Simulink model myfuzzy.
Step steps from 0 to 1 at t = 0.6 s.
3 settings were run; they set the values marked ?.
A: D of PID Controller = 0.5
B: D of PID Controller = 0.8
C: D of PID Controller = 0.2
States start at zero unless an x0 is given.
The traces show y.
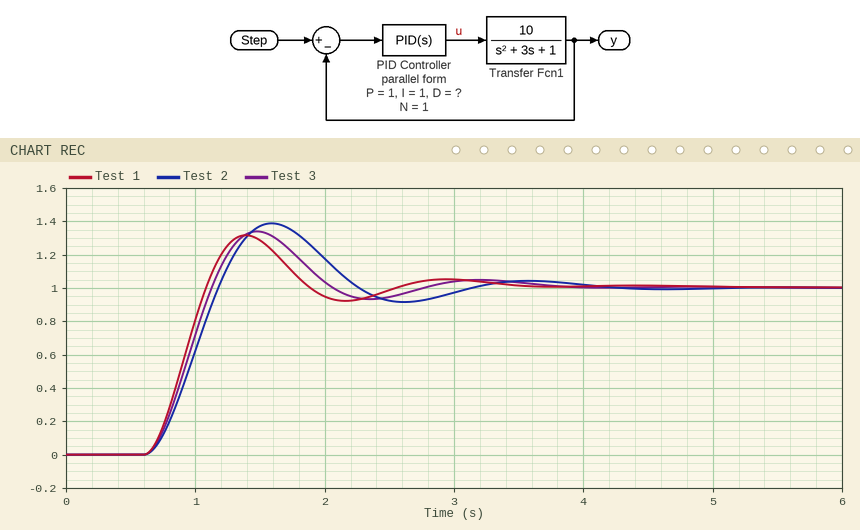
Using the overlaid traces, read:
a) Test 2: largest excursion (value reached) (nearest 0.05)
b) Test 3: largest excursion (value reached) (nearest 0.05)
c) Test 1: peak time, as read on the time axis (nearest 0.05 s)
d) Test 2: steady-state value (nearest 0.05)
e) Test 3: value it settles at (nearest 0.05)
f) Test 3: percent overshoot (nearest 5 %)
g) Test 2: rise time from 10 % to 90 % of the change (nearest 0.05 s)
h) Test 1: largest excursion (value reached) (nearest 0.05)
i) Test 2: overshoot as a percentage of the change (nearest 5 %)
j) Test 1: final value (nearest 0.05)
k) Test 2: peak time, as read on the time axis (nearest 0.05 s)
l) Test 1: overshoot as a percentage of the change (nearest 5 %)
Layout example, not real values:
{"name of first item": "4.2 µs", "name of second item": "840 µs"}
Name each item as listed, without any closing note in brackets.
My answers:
{"Test 2: largest excursion (value reached)": "1.40", "Test 3: largest excursion (value reached)": "1.35", "Test 1: peak time, as read on the time axis": "1.40 s", "Test 2: steady-state value": "1.00", "Test 3: value it settles at": "1.00", "Test 3: percent overshoot": "35 %", "Test 2: rise time from 10 % to 90 % of the change": "0.40 s", "Test 1: largest excursion (value reached)": "1.30", "Test 2: overshoot as a percentage of the change": "40 %", "Test 1: final value": "1.00", "Test 2: peak time, as read on the time axis": "1.60 s", "Test 1: overshoot as a percentage of the change": "30 %"}
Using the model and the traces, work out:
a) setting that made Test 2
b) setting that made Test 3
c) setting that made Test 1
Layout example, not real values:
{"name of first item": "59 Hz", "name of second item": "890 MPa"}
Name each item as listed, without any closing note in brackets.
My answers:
{"setting that made Test 2": "C", "setting that made Test 3": "A", "setting that made Test 1": "B"}
